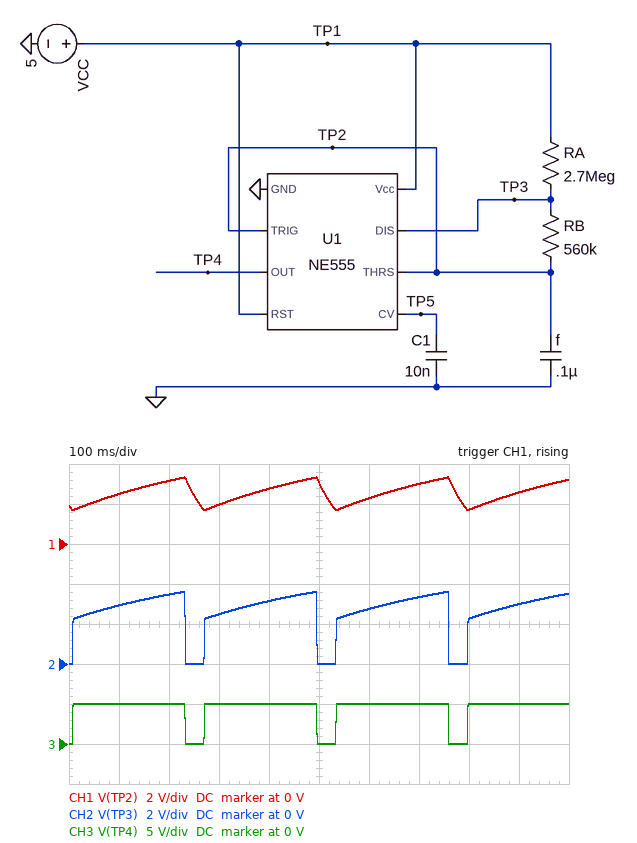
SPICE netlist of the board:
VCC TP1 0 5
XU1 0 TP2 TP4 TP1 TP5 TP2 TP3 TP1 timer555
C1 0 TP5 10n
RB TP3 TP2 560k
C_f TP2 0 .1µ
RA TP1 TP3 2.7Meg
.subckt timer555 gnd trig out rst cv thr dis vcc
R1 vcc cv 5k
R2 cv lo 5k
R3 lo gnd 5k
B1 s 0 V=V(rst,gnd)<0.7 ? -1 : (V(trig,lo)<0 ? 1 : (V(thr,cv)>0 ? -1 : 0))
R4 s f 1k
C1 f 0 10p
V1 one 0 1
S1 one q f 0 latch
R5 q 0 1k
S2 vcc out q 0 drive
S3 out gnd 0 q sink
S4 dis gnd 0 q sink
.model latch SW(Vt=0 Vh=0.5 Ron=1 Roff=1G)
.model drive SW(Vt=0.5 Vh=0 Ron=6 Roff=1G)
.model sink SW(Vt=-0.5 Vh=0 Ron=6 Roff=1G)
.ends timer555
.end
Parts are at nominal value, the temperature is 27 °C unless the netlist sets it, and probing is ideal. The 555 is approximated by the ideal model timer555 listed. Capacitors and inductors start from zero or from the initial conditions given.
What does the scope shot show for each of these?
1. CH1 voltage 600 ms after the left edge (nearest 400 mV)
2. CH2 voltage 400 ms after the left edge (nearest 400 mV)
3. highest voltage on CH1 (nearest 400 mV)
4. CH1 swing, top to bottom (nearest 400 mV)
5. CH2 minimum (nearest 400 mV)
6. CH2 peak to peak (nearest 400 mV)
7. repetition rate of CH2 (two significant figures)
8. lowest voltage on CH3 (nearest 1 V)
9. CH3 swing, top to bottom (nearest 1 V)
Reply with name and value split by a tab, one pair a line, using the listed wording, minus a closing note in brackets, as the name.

CH1 voltage 600 ms after the left edge	2.4 V
CH2 voltage 400 ms after the left edge	3.2 V
highest voltage on CH1	3.2 V
CH1 swing, top to bottom	1.6 V
CH2 minimum	0 V
CH2 peak to peak	3.6 V
repetition rate of CH2	3.8 Hz
lowest voltage on CH3	0 V
CH3 swing, top to bottom	5 V
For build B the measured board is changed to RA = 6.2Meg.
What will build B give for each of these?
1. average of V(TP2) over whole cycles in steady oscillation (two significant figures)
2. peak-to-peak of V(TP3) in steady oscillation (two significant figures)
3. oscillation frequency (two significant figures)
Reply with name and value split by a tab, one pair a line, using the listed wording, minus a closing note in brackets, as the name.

average of V(TP2) over whole cycles in steady oscillation	2.6 V
peak-to-peak of V(TP3) in steady oscillation	3.5 V
oscillation frequency	2.0 Hz
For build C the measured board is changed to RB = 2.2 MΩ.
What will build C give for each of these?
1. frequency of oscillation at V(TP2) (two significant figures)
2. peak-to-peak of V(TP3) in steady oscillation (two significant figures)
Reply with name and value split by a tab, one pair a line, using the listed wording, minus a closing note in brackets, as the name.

frequency of oscillation at V(TP2)	2.0 Hz
peak-to-peak of V(TP3) in steady oscillation	4.1 V
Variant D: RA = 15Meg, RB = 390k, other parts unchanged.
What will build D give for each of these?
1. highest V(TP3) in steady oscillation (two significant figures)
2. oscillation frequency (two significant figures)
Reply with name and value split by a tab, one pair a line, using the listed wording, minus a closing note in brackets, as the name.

highest V(TP3) in steady oscillation	3.4 V
oscillation frequency	900 mHz
